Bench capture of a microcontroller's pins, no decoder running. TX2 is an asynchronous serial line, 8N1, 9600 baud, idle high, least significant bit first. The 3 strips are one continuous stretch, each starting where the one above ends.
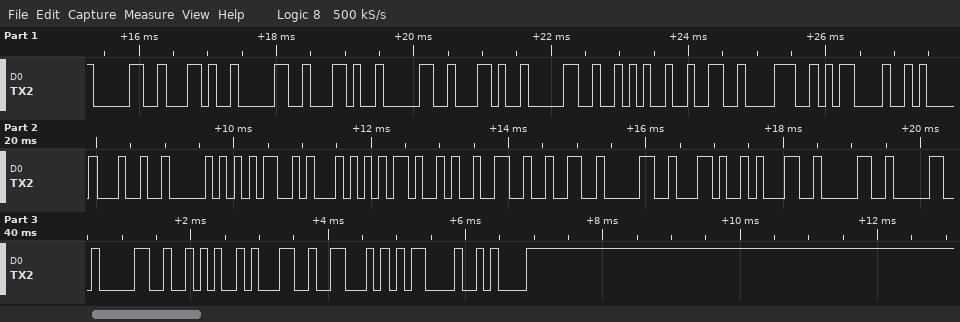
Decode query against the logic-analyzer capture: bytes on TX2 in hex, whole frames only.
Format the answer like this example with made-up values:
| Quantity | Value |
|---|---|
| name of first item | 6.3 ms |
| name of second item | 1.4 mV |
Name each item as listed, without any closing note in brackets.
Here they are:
| Quantity | Value |
|---|---|
| bytes on TX2 in hex, whole frames only | 30 2C 30 2C 30 2C 30 2A 32 38 0D 0A 24 50 4D 54 4B 32 32 30 2C 31 30 30 30 2A 31 46 0D 0A |
